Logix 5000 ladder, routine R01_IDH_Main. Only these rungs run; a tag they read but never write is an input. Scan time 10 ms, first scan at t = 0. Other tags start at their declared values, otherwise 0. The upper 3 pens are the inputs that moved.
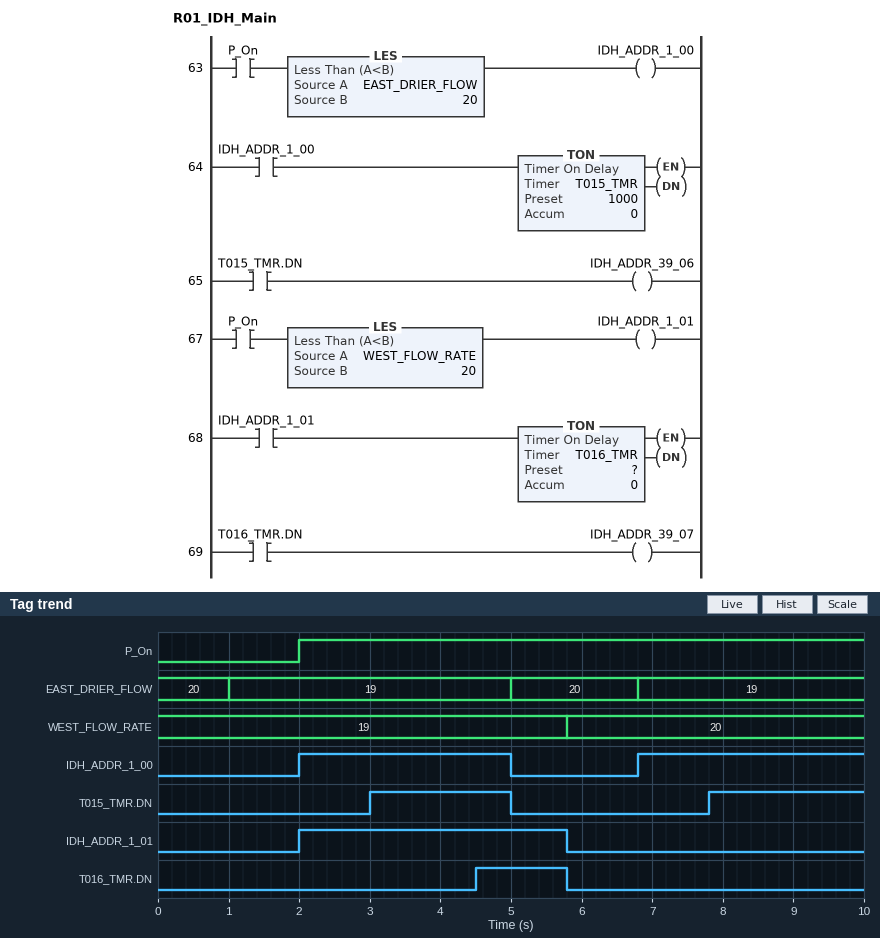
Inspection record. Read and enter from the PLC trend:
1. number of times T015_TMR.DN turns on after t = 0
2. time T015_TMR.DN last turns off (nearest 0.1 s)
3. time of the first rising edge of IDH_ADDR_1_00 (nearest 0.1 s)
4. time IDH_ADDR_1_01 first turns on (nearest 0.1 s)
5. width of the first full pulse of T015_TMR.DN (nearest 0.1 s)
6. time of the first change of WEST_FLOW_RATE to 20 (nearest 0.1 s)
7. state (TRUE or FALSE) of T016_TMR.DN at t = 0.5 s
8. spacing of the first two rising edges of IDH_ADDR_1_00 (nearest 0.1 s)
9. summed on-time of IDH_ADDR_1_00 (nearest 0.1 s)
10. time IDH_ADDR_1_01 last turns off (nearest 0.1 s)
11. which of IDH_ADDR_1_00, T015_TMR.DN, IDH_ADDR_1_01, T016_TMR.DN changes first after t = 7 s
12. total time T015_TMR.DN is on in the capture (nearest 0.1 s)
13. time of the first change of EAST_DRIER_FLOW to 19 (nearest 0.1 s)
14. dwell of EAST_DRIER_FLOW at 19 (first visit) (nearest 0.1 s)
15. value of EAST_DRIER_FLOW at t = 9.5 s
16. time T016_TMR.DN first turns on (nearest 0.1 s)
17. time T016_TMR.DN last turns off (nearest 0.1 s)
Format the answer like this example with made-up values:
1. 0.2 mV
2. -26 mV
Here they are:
1. 2
2. 5.0 s
3. 2.0 s
4. 2.0 s
5. 2.0 s
6. 5.8 s
7. FALSE
8. 4.8 s
9. 6.2 s
10. 5.8 s
11. T015_TMR.DN
12. 4.2 s
13. 1.0 s
14. 4.0 s
15. 19
16. 4.5 s
17. 5.8 s
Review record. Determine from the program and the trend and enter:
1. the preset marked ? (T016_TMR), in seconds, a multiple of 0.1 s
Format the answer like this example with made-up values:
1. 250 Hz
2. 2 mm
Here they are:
1. 2.5 s
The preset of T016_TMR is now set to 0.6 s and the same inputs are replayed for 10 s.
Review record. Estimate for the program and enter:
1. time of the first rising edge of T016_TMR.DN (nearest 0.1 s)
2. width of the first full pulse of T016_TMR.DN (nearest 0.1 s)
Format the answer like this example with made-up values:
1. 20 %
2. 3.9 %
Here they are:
1. 2.6 s
2. 3.2 s
